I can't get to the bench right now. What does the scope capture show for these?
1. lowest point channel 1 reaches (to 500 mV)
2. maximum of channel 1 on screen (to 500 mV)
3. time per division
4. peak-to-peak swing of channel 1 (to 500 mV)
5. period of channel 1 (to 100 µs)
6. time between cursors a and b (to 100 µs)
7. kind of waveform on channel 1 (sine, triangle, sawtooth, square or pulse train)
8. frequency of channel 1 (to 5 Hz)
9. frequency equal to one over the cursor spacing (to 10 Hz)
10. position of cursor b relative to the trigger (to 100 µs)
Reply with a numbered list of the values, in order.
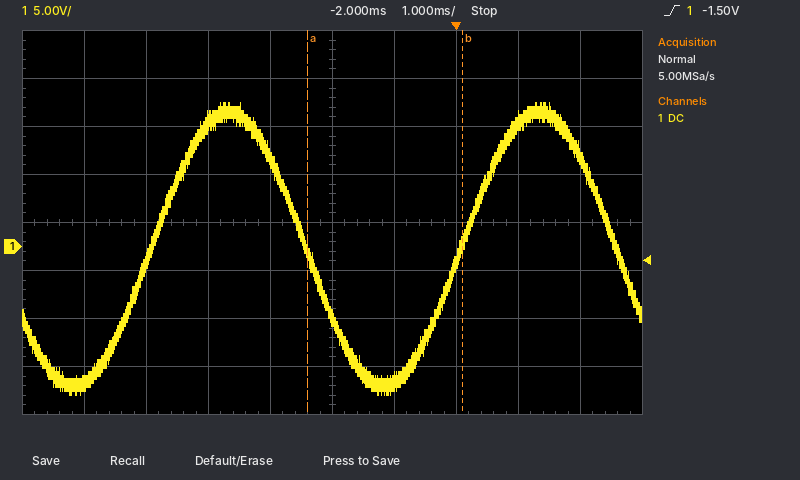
1. -15.5 V
2. 15.0 V
3. 1 ms
4. 30.5 V
5. 5.0 ms
6. 2.5 ms
7. sine
8. 200 Hz
9. 400 Hz
10. +100 µs
